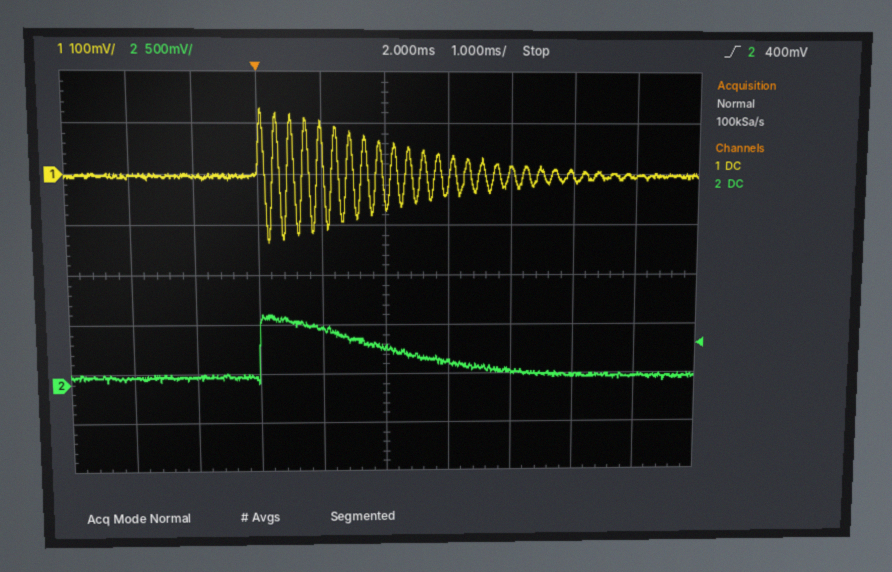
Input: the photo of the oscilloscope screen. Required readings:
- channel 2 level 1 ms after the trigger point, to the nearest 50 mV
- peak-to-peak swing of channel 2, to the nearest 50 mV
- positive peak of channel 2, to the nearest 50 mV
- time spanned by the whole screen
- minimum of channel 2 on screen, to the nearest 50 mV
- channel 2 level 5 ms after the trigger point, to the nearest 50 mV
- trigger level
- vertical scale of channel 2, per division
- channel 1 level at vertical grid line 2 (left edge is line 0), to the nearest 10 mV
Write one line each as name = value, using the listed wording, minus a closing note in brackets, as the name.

channel 2 level 1 ms after the trigger point, to the nearest 50 mV = 550 mV
peak-to-peak swing of channel 2, to the nearest 50 mV = 700 mV
positive peak of channel 2, to the nearest 50 mV = 700 mV
time spanned by the whole screen = 10 ms
minimum of channel 2 on screen, to the nearest 50 mV = 0 mV
channel 2 level 5 ms after the trigger point, to the nearest 50 mV = 100 mV
trigger level = 400 mV
vertical scale of channel 2, per division = 500 mV
channel 1 level at vertical grid line 2 (left edge is line 0), to the nearest 10 mV = 0 mV
